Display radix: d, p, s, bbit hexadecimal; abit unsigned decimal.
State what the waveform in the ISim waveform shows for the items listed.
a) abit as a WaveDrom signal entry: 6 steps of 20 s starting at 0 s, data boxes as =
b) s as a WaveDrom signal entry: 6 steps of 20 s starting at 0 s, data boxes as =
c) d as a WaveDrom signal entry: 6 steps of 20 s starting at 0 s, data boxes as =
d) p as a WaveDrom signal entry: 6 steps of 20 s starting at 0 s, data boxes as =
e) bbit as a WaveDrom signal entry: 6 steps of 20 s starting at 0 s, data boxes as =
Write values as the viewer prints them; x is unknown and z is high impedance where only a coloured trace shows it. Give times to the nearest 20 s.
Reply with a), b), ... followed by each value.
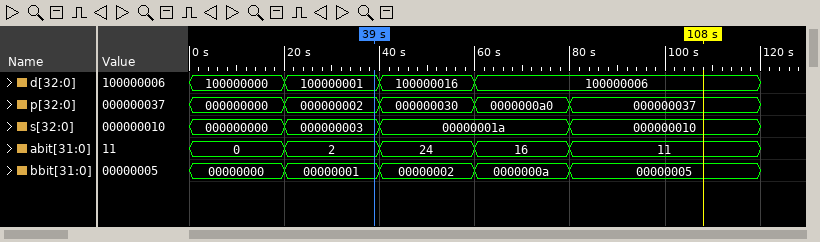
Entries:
a) {name: 'abit', wave: '=====.', data: '0 2 24 16 11'}
b) {name: 's', wave: '===.=.', data: '000000000 000000003 00000001a 000000010'}
c) {name: 'd', wave: '====..', data: '100000000 100000001 100000016 100000006'}
d) {name: 'p', wave: '=====.', data: '000000000 000000002 000000030 0000000a0 000000037'}
e) {name: 'bbit', wave: '=====.', data: '00000000 00000001 00000002 0000000a 00000005'}
